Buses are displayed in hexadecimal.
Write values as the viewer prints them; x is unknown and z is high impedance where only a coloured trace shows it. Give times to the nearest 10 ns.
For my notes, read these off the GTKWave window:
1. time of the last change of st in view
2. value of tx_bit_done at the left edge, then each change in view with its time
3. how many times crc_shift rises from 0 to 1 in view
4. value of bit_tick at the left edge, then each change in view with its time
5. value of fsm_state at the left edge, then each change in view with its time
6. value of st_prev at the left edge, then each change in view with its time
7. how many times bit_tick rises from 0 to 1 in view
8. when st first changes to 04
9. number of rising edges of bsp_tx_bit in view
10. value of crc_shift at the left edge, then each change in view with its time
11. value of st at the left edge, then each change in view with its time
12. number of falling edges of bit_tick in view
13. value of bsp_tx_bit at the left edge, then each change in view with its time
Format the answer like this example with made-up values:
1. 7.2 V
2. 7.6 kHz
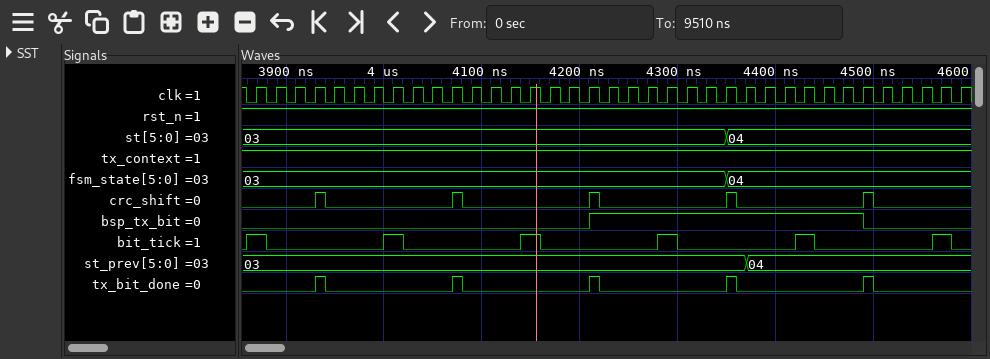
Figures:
1. 4350 ns
2. 0, 1 at 3930 ns, 0 at 3940 ns, 1 at 4070 ns, 0 at 4080 ns, 1 at 4210 ns, 0 at 4220 ns, 1 at 4350 ns, 0 at 4360 ns, 1 at 4490 ns, 0 at 4500 ns
3. 5
4. 0, 1 at 3860 ns, 0 at 3880 ns, 1 at 4000 ns, 0 at 4020 ns, 1 at 4140 ns, 0 at 4160 ns, 1 at 4280 ns, 0 at 4300 ns, 1 at 4420 ns, 0 at 4440 ns, 1 at 4560 ns, 0 at 4580 ns
5. 03, 04 at 4350 ns
6. 03, 04 at 4370 ns
7. 6
8. 4350 ns
9. 1
10. 0, 1 at 3930 ns, 0 at 3940 ns, 1 at 4070 ns, 0 at 4080 ns, 1 at 4210 ns, 0 at 4220 ns, 1 at 4350 ns, 0 at 4360 ns, 1 at 4490 ns, 0 at 4500 ns
11. 03, 04 at 4350 ns
12. 6
13. 0, 1 at 4210 ns, 0 at 4490 ns
